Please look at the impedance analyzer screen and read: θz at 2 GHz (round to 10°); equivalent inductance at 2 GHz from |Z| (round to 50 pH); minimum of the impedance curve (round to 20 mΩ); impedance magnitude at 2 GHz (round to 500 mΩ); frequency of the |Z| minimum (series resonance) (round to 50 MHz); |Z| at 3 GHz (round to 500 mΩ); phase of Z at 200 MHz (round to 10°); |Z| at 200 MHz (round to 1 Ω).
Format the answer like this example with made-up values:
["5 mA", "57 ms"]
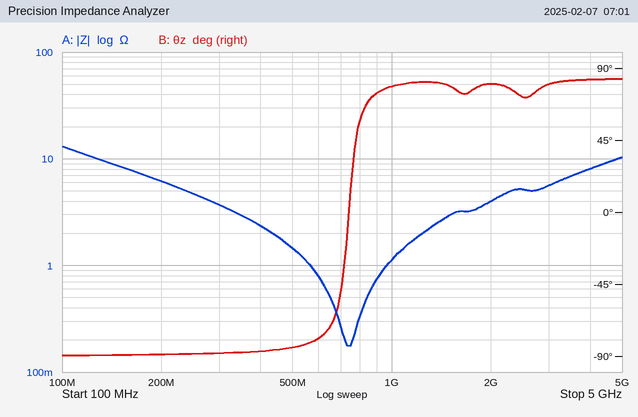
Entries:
["80°", "300 pH", "180 mΩ", "4.0 Ω", "750 MHz", "5.5 Ω", "-90°", "6 Ω"]
